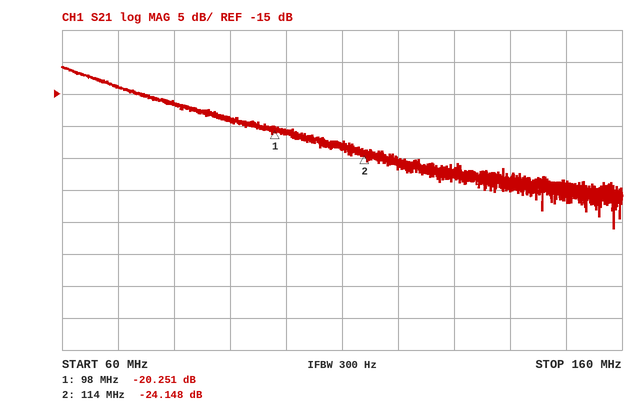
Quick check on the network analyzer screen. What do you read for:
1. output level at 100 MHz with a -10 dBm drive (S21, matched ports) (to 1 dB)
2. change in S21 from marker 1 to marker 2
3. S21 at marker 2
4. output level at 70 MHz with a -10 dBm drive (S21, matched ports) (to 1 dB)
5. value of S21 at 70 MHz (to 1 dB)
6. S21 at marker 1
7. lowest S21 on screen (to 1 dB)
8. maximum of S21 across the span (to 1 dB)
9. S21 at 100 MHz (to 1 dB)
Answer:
-31 dBm
-3.897 dB
-24.148 dB
-24 dBm
-14 dB
-20.251 dB
-36 dB
-11 dB
-21 dB
